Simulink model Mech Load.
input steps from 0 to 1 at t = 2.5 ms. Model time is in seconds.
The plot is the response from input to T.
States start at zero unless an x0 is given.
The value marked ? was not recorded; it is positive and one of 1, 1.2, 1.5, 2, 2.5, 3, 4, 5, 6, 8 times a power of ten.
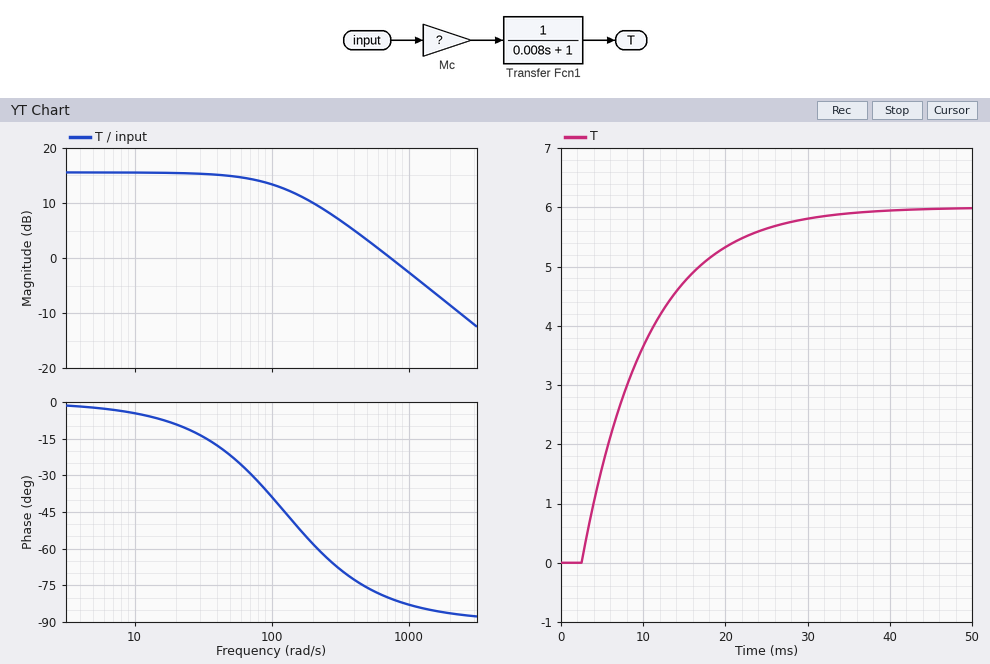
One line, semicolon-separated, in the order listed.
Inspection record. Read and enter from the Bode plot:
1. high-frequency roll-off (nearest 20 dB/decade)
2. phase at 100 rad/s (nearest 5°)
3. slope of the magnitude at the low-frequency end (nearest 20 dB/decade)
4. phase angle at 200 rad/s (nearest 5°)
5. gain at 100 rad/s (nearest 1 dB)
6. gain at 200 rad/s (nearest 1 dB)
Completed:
-20 dB/decade; -40°; 0 dB/decade; -60°; 13 dB; 10 dB
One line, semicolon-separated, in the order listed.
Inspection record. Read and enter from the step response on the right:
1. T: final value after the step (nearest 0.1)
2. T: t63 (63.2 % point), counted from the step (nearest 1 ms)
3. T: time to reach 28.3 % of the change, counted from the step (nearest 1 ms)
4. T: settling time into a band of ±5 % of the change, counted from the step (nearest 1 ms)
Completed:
6.0; 8 ms; 3 ms; 24 ms
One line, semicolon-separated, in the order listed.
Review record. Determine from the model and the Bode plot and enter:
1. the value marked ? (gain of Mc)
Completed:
6
